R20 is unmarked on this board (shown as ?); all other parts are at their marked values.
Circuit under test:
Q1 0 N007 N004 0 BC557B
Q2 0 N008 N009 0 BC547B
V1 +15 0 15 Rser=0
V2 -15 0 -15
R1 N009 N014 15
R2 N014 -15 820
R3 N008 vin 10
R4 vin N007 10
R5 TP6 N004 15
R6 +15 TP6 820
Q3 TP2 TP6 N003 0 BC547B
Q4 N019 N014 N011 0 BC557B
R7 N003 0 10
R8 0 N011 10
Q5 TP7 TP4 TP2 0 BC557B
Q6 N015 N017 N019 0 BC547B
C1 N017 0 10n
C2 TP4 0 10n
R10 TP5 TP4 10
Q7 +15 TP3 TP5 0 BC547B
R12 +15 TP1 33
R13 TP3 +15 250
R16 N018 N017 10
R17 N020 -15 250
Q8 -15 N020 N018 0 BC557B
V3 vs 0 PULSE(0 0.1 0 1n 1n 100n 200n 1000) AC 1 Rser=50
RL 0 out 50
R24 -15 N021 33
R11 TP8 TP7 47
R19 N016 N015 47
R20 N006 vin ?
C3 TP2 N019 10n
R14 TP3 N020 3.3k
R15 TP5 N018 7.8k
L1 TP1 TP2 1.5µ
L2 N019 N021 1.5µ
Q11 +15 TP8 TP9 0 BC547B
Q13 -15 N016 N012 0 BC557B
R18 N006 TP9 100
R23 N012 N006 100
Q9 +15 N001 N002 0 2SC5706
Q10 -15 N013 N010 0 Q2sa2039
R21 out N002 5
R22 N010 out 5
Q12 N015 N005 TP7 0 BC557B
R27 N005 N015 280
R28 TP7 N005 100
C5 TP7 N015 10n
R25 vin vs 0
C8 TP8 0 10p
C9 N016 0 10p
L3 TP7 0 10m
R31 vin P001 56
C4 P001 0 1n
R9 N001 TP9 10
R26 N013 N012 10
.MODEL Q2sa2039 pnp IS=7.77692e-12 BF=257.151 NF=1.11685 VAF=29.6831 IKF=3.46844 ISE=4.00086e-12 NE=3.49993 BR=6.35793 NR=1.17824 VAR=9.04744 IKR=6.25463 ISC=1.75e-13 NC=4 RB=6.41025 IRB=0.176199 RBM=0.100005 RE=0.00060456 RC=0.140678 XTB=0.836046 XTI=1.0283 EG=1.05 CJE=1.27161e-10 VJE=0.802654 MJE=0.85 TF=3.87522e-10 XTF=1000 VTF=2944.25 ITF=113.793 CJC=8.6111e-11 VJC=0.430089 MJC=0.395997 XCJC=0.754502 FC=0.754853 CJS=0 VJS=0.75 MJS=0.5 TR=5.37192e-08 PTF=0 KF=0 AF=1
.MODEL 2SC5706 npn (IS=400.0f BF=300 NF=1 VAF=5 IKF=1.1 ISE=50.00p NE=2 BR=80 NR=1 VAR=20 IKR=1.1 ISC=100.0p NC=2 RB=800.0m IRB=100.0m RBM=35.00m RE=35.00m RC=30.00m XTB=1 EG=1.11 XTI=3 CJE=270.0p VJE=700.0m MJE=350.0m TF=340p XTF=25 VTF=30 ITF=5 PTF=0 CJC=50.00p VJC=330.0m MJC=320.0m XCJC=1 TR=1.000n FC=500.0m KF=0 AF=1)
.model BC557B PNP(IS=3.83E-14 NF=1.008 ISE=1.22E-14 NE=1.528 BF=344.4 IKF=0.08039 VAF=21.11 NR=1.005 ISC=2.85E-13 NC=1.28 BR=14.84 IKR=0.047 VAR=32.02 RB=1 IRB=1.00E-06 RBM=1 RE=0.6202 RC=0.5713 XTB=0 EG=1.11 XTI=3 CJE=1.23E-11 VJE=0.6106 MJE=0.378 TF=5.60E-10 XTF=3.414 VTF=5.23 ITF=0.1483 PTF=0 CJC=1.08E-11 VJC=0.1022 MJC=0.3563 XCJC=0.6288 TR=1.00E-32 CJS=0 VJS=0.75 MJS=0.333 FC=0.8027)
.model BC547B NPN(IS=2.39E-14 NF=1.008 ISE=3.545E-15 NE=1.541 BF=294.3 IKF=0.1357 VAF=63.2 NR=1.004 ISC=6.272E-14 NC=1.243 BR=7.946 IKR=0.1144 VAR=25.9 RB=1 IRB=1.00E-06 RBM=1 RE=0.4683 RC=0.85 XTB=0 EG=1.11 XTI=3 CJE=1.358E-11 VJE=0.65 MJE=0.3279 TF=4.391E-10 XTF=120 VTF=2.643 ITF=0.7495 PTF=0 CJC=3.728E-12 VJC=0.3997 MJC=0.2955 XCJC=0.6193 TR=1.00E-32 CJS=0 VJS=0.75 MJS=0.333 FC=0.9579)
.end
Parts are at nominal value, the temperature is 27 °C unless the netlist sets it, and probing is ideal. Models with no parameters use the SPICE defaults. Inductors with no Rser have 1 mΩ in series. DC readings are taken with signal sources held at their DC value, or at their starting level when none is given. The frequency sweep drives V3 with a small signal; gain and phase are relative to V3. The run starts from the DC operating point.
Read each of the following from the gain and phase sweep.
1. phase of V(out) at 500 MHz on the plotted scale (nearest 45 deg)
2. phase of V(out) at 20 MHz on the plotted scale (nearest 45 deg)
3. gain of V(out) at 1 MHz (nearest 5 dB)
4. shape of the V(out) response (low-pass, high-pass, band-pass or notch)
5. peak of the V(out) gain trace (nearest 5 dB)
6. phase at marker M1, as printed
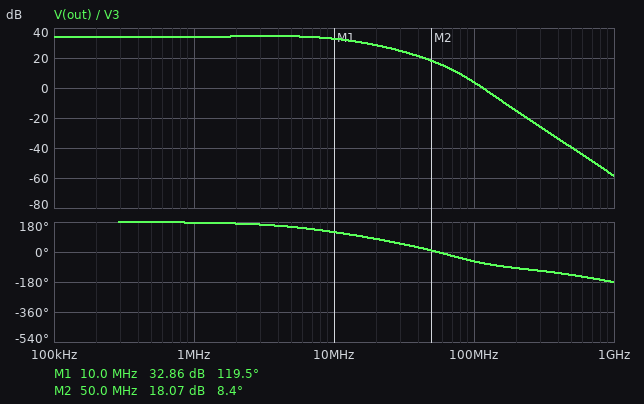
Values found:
-135 deg
90 deg
35 dB
low-pass
35 dB
119.5 deg
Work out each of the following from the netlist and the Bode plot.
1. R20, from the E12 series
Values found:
2.7 kΩ
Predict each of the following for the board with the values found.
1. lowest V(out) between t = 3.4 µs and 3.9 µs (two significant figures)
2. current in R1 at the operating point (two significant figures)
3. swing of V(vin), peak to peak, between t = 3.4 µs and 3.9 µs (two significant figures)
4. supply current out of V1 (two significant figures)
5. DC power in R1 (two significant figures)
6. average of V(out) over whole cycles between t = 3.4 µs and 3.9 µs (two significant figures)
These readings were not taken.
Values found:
-6.3 V
17 mA
110 mV
100 mA
4.3 mW
-3.5 V
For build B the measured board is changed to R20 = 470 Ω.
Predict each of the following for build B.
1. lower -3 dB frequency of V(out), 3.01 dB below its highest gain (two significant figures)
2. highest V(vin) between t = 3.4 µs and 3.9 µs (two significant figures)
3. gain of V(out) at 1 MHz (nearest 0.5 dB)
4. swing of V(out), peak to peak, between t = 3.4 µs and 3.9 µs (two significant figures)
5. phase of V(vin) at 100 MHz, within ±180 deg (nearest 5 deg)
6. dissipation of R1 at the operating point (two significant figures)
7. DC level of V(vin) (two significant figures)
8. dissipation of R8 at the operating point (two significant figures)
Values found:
29 MHz
-72 mV
19.5 dB
1.9 V
-50 deg
4.3 mW
-120 mV
13 mW
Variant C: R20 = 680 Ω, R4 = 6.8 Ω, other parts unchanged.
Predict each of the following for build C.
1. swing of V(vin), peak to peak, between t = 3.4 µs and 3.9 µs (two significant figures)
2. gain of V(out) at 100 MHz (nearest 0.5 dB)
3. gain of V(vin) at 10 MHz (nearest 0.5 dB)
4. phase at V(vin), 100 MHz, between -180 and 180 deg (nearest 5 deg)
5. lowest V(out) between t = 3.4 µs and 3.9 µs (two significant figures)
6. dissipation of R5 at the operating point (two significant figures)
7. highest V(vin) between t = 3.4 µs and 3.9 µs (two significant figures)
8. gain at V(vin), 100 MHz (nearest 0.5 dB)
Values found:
97 mV
2.5 dB
-15.0 dB
-50 deg
-3.0 V
4.4 mW
-36 mV
-8.0 dB
